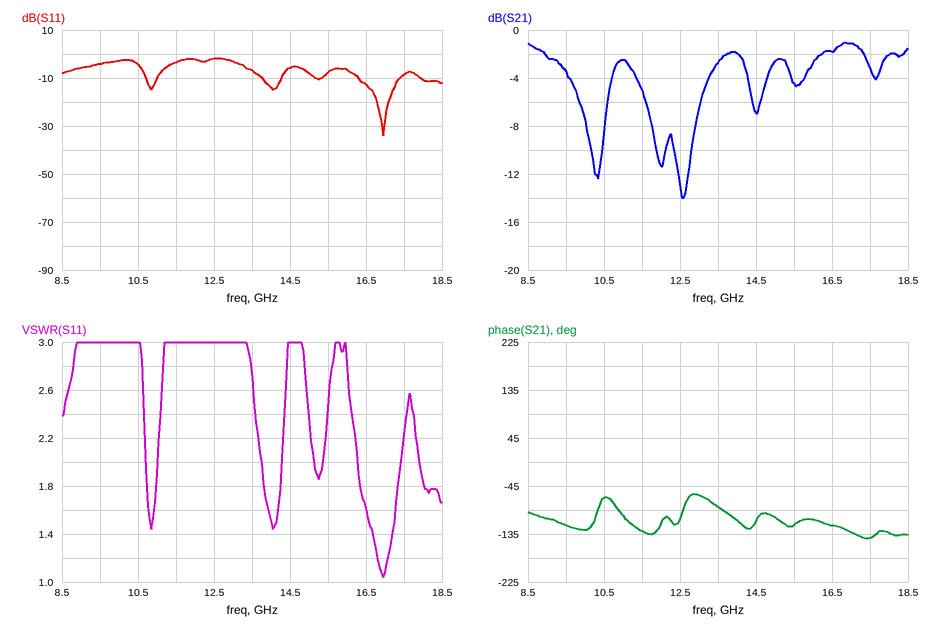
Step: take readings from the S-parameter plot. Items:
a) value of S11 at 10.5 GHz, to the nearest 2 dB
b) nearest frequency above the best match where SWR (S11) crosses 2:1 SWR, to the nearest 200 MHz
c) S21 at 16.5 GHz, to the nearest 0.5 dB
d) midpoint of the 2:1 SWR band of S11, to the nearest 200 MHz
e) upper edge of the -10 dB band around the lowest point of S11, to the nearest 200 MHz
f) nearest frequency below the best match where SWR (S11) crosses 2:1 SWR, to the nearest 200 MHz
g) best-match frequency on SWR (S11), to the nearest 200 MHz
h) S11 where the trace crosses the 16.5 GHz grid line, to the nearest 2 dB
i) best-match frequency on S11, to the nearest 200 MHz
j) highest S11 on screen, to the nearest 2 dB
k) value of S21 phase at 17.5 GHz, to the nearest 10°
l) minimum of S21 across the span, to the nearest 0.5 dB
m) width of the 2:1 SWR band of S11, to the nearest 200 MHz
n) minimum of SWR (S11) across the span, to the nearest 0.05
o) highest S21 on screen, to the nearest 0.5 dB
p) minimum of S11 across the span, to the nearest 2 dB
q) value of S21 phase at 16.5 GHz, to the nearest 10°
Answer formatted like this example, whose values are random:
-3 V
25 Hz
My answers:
-4 dB
17.4 GHz
-2.0 dB
16.8 GHz
17.4 GHz
16.2 GHz
17.0 GHz
-12 dB
17.0 GHz
-2 dB
-140°
-14.0 dB
1.2 GHz
1.05
-1.0 dB
-34 dB
-120°
